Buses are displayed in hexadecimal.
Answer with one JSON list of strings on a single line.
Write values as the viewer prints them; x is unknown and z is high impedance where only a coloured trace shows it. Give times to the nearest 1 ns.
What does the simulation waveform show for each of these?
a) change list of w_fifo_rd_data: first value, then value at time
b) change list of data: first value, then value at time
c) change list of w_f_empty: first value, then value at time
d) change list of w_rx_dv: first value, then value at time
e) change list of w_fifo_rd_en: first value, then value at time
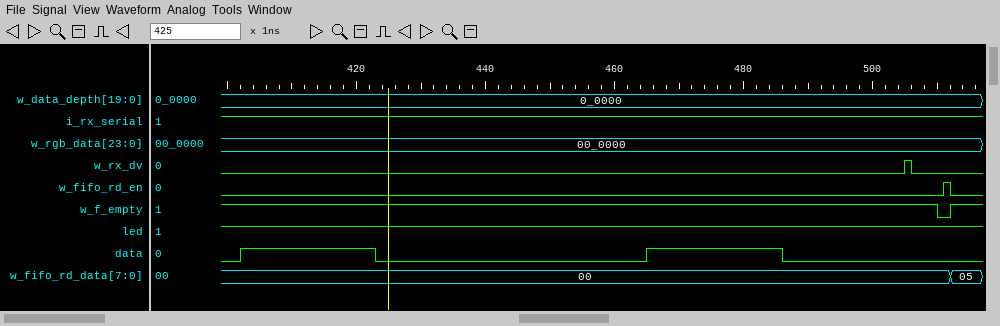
["00, 05 at 512 ns", "0, 1 at 402 ns, 0 at 423 ns, 1 at 465 ns, 0 at 486 ns", "1, 0 at 510 ns, 1 at 512 ns", "0, 1 at 505 ns, 0 at 506 ns", "0, 1 at 511 ns, 0 at 512 ns"]
